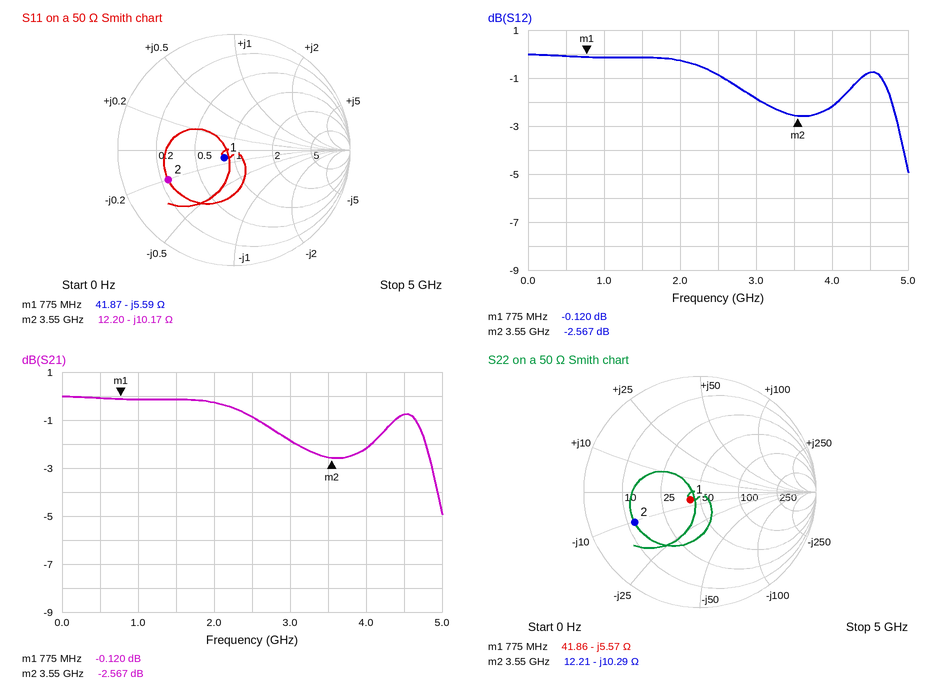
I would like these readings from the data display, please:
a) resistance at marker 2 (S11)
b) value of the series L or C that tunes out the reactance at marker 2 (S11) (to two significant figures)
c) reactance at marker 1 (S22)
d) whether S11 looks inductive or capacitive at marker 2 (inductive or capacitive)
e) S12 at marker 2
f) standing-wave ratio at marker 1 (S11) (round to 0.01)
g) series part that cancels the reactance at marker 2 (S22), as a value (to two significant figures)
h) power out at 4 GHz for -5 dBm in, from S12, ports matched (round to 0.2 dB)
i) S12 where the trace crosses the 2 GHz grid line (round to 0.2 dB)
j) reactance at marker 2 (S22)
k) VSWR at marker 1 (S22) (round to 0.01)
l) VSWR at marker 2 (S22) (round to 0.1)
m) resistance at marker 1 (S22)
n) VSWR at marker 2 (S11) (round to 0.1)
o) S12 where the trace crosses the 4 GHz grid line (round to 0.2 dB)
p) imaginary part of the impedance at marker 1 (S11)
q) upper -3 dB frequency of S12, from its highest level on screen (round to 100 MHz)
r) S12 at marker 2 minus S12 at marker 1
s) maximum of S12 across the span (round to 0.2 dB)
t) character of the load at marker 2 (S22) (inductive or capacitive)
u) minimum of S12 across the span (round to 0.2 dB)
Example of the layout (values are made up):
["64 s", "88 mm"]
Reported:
["12.20 Ω", "460 pH", "-5.57 Ω", "capacitive", "-2.567 dB", "1.24", "460 pH", "-7.2 dBm", "-0.2 dB", "-10.29 Ω", "1.24", "4.3", "41.86 Ω", "4.3", "-2.2 dB", "-5.59 Ω", "4.9 GHz", "-2.447 dB", "0.0 dB", "capacitive", "-5.0 dB"]
